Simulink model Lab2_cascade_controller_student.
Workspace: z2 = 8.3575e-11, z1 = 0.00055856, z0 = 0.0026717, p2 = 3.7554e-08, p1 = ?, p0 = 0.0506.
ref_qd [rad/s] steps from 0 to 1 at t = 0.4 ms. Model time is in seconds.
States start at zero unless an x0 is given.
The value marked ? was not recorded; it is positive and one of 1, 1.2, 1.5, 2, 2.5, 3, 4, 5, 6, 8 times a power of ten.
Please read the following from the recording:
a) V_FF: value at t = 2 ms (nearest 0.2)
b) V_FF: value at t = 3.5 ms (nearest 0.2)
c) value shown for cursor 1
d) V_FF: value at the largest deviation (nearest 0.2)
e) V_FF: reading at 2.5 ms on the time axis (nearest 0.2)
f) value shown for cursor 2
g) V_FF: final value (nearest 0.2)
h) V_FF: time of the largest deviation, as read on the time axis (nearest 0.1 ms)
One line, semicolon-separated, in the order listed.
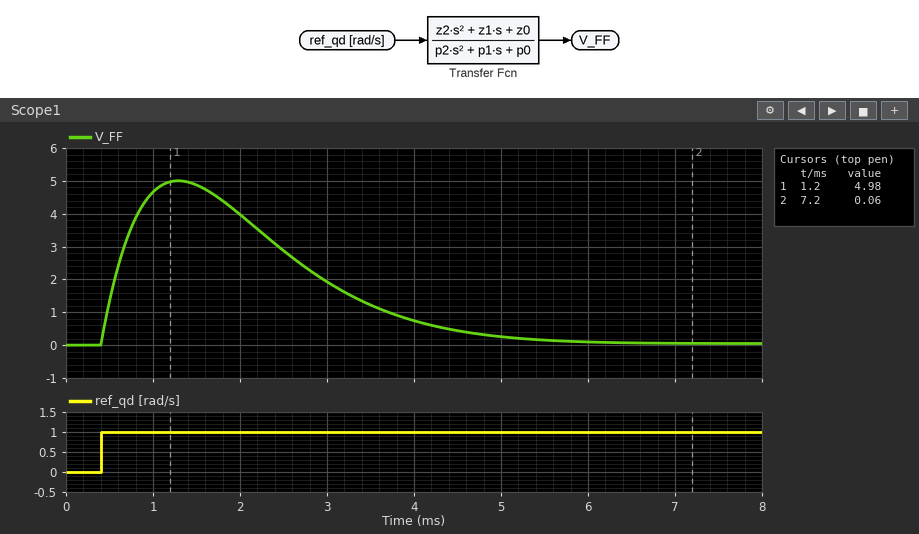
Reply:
4.0; 1.2; 4.98; 5.0; 2.8; 0.06; 0.0; 1.3 ms
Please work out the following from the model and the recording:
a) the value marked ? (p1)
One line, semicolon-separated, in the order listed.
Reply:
8e-05
